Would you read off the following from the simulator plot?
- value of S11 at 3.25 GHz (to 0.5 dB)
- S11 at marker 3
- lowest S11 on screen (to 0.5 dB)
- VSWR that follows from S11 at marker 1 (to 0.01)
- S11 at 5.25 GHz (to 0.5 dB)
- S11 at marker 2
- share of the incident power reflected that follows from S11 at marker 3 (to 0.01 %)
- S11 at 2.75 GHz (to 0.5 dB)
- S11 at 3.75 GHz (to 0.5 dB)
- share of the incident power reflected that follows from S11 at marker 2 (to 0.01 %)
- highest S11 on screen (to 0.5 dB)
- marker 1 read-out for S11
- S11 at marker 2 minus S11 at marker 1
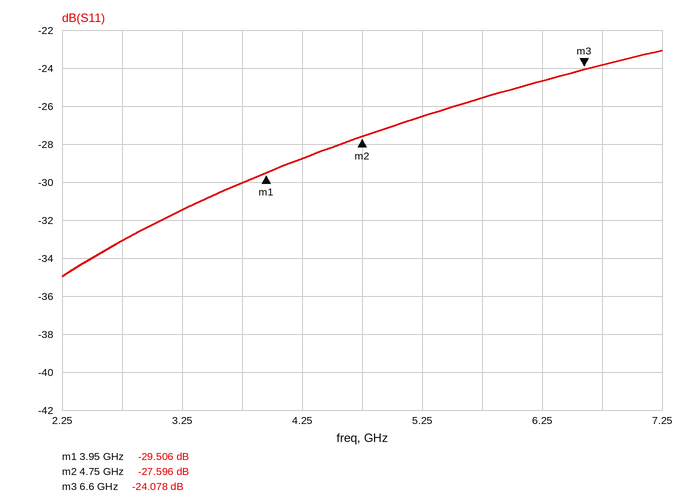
-31.5 dB
-24.078 dB
-35.0 dB
1.07
-26.5 dB
-27.596 dB
0.39 %
-33.0 dB
-30.0 dB
0.17 %
-23.0 dB
-29.506 dB
1.910 dB
